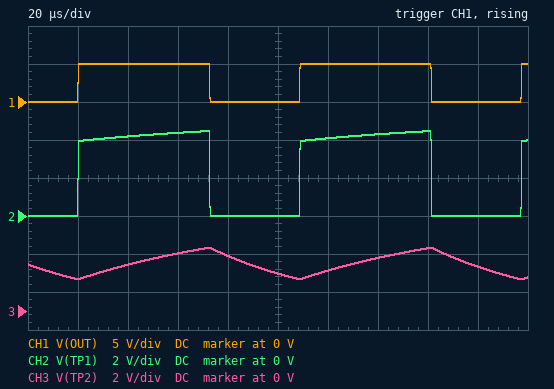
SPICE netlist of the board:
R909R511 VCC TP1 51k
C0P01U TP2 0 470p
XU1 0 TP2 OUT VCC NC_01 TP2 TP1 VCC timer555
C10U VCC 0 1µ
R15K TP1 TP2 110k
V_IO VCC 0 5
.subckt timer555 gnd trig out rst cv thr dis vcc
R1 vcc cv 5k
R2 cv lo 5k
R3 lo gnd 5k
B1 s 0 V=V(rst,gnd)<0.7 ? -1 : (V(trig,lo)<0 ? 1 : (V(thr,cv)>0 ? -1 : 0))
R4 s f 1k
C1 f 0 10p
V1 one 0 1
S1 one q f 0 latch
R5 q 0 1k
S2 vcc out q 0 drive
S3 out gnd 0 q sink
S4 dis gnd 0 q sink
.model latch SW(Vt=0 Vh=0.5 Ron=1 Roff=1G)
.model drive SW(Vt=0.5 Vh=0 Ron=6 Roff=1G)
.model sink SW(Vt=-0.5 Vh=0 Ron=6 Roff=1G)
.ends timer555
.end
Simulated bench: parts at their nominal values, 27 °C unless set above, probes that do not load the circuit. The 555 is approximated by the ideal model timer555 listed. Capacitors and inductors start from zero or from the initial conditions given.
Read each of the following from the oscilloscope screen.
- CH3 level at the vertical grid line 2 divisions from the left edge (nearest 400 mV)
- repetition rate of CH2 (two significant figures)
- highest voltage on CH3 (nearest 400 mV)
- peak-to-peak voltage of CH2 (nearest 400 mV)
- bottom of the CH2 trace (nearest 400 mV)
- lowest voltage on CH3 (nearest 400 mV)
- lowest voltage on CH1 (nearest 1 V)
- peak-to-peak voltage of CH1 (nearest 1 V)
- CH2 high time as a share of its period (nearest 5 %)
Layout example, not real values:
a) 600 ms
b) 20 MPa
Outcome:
a) 2.4 V
b) 11 kHz
c) 3.2 V
d) 4.4 V
e) 0 V
f) 1.6 V
g) 0 V
h) 5 V
i) 60 %
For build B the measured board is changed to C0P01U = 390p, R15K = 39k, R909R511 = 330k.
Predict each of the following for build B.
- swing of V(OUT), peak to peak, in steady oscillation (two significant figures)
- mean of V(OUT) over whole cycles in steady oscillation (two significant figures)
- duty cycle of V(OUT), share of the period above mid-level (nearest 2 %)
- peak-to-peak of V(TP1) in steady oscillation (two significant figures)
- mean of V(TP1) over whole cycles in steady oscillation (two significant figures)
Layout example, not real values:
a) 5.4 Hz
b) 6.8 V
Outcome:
a) 5.0 V
b) 4.5 V
c) 90 %
d) 3.5 V
e) 2.6 V
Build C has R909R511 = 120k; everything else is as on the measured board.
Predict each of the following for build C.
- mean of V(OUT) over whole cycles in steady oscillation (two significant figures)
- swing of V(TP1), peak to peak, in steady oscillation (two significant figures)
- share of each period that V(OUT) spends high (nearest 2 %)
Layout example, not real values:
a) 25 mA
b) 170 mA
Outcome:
a) 3.4 V
b) 4.1 V
c) 68 %
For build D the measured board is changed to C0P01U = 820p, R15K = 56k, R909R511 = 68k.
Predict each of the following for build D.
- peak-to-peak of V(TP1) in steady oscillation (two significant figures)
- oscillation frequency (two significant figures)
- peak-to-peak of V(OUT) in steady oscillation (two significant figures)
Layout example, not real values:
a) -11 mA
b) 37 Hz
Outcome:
a) 4.1 V
b) 9.8 kHz
c) 5.0 V
